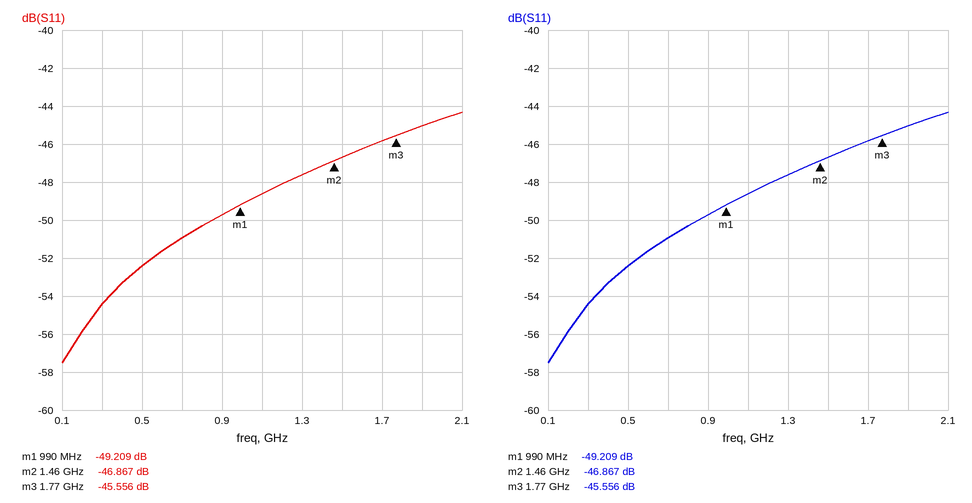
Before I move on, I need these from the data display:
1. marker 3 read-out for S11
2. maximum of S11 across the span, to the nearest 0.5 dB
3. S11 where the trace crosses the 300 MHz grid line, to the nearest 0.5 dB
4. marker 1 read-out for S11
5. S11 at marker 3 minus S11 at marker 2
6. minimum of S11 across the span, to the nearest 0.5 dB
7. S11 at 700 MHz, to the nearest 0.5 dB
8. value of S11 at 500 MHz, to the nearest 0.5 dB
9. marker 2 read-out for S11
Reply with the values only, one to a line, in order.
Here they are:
-45.556 dB
-44.5 dB
-54.5 dB
-49.209 dB
1.311 dB
-57.5 dB
-51.0 dB
-52.5 dB
-46.867 dB
